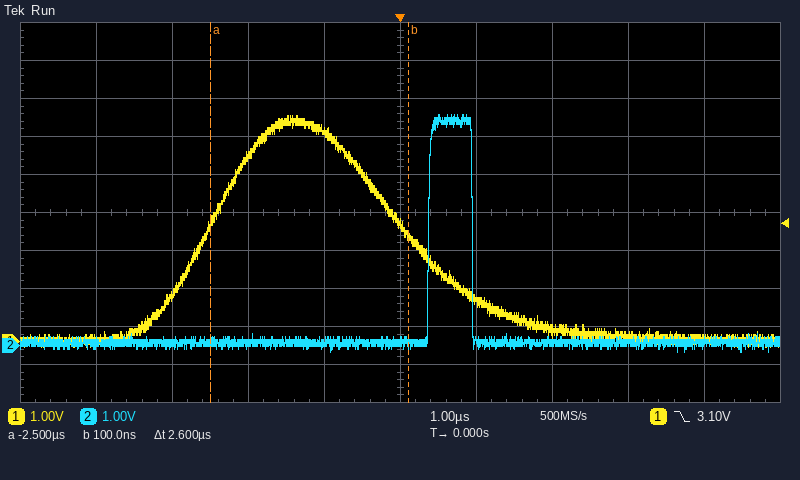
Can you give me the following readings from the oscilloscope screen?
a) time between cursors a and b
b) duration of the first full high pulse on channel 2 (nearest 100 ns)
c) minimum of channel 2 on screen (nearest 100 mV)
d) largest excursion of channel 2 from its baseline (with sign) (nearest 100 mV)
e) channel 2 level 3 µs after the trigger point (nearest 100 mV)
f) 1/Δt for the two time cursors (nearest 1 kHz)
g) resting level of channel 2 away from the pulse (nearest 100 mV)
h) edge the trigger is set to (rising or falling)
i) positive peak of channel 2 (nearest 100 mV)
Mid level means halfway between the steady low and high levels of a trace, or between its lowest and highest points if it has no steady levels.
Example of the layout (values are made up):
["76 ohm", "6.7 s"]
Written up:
["2.6 µs", "600 ns", "-200 mV", "+6.0 V", "100 mV", "385 kHz", "100 mV", "falling", "6.1 V"]
